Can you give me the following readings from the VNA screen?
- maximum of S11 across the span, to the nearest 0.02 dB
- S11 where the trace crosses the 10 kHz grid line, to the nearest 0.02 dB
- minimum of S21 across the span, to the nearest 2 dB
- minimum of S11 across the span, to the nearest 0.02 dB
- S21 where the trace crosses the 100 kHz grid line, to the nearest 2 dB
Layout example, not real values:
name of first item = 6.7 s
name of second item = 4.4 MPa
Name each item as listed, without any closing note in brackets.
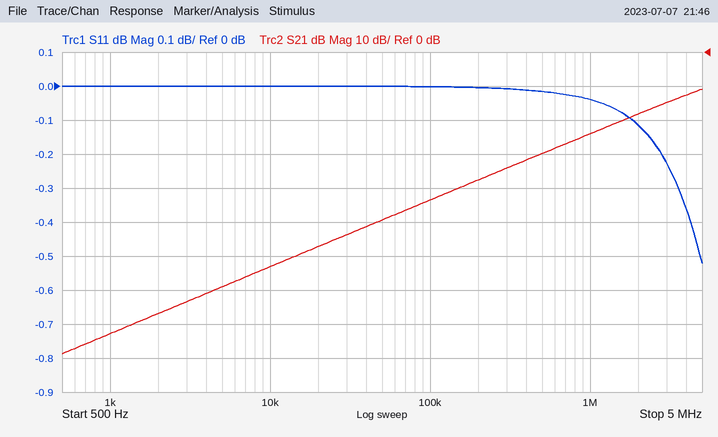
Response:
maximum of S11 across the span, to the nearest 0.02 dB = 0.00 dB
S11 where the trace crosses the 10 kHz grid line, to the nearest 0.02 dB = 0.00 dB
minimum of S21 across the span, to the nearest 2 dB = -88 dB
minimum of S11 across the span, to the nearest 0.02 dB = -0.52 dB
S21 where the trace crosses the 100 kHz grid line, to the nearest 2 dB = -44 dB
